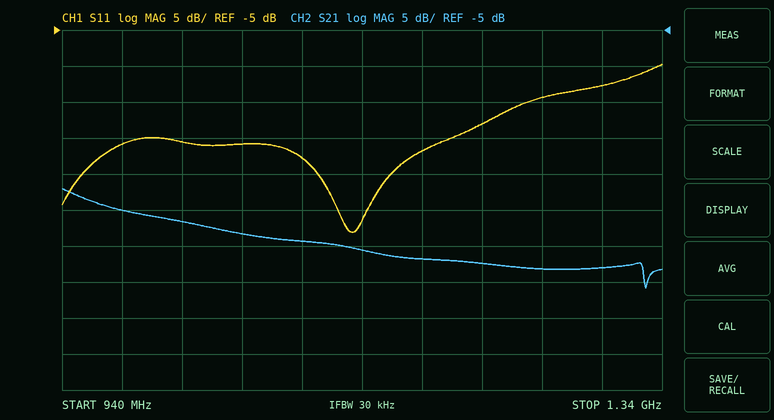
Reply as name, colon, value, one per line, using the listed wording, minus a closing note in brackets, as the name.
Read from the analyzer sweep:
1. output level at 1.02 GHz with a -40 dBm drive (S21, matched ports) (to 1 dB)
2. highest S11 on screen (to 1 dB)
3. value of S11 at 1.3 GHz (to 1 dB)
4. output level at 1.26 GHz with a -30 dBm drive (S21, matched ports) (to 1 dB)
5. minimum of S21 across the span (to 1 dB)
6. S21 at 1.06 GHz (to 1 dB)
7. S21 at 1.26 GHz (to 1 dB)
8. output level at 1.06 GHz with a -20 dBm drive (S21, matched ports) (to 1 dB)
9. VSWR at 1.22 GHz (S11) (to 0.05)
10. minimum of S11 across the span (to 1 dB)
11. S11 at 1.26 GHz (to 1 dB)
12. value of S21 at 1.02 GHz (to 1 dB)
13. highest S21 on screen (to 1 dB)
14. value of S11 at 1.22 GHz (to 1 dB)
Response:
output level at 1.02 GHz with a -40 dBm drive (S21, matched ports): -72 dBm
highest S11 on screen: -10 dB
value of S11 at 1.3 GHz: -13 dB
output level at 1.26 GHz with a -30 dBm drive (S21, matched ports): -68 dBm
minimum of S21 across the span: -41 dB
S21 at 1.06 GHz: -33 dB
S21 at 1.26 GHz: -38 dB
output level at 1.06 GHz with a -20 dBm drive (S21, matched ports): -53 dBm
VSWR at 1.22 GHz (S11): 1.30
minimum of S11 across the span: -33 dB
S11 at 1.26 GHz: -14 dB
value of S21 at 1.02 GHz: -32 dB
highest S21 on screen: -27 dB
value of S11 at 1.22 GHz: -18 dB
